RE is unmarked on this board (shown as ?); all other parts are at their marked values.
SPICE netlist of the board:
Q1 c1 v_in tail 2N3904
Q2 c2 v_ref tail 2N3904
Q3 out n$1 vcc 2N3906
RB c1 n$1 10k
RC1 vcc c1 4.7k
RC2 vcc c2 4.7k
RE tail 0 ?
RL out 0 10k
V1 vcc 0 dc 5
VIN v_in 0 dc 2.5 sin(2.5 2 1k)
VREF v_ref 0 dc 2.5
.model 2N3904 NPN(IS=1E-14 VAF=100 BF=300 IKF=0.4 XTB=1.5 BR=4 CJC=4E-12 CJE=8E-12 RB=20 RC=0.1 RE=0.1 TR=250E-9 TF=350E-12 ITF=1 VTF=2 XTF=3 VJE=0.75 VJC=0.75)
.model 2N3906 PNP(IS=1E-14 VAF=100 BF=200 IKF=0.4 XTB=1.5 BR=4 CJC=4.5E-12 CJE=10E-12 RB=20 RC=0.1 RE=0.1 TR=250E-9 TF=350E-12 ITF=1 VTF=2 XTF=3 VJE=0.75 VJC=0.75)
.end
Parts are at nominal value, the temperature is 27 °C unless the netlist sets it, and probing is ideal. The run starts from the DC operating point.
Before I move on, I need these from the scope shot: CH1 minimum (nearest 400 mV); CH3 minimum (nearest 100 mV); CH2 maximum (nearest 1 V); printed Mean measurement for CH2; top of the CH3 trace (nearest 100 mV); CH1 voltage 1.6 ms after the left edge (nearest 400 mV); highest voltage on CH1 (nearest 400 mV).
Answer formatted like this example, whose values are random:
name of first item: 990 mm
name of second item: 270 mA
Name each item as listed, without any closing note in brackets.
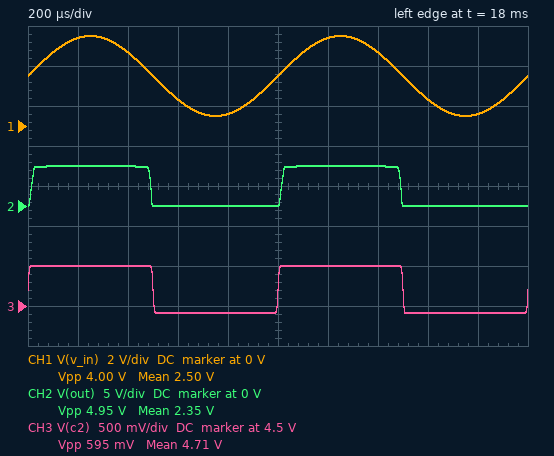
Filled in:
CH1 minimum: 400 mV
CH3 minimum: 4.4 V
CH2 maximum: 5 V
printed Mean measurement for CH2: 2.35 V
top of the CH3 trace: 5.0 V
CH1 voltage 1.6 ms after the left edge: 1.2 V
highest voltage on CH1: 4.4 V
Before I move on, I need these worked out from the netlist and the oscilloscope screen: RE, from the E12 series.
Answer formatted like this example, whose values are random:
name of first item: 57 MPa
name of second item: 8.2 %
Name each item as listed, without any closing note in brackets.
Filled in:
RE, from the E12 series: 15 kΩ
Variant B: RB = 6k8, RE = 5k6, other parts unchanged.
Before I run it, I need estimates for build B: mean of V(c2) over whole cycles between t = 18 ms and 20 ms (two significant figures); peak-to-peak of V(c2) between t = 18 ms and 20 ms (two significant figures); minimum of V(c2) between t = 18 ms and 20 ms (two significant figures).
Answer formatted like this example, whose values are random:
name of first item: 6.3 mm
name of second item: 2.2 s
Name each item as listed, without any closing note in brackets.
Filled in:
mean of V(c2) over whole cycles between t = 18 ms and 20 ms: 4.2 V
peak-to-peak of V(c2) between t = 18 ms and 20 ms: 1.6 V
minimum of V(c2) between t = 18 ms and 20 ms: 3.4 V
